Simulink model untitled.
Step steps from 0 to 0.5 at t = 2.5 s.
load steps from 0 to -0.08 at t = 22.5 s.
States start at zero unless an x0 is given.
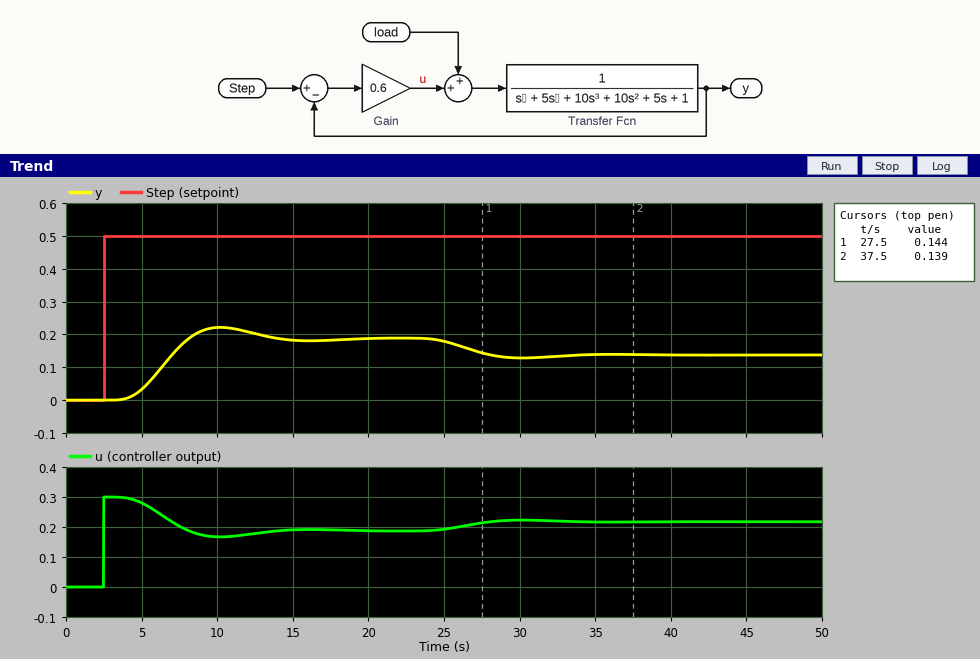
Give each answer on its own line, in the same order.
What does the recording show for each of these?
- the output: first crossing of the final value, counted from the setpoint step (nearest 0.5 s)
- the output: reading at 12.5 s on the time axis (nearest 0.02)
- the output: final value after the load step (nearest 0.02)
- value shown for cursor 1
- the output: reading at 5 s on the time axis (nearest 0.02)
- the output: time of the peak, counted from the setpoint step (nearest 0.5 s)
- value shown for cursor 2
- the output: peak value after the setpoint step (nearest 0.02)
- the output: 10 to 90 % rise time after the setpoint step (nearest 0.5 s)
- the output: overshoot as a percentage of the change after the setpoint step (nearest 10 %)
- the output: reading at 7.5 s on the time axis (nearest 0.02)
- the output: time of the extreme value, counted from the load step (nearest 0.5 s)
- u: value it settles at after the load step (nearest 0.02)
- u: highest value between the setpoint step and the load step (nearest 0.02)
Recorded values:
5.5 s
0.20
0.14
0.144
0.04
7.5 s
0.139
0.22
3.0 s
20 %
0.16
7.5 s
0.22
0.30
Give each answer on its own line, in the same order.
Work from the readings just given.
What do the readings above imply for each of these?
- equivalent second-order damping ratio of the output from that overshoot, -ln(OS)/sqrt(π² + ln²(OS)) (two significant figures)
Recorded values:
0.46
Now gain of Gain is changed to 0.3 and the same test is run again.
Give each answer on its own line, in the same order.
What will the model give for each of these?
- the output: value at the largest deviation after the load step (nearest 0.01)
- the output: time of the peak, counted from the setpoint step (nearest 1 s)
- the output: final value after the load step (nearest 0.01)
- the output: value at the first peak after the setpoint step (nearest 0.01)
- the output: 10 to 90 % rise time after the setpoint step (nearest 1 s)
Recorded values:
0.05
9 s
0.05
0.12
4 s
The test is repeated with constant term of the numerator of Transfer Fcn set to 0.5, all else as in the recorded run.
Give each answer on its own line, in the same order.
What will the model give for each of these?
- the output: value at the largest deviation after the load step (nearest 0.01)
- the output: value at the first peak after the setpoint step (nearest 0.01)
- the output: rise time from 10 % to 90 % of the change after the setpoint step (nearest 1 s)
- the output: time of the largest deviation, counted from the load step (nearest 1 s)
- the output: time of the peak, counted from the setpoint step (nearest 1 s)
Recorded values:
0.08
0.12
4 s
9 s
9 s
